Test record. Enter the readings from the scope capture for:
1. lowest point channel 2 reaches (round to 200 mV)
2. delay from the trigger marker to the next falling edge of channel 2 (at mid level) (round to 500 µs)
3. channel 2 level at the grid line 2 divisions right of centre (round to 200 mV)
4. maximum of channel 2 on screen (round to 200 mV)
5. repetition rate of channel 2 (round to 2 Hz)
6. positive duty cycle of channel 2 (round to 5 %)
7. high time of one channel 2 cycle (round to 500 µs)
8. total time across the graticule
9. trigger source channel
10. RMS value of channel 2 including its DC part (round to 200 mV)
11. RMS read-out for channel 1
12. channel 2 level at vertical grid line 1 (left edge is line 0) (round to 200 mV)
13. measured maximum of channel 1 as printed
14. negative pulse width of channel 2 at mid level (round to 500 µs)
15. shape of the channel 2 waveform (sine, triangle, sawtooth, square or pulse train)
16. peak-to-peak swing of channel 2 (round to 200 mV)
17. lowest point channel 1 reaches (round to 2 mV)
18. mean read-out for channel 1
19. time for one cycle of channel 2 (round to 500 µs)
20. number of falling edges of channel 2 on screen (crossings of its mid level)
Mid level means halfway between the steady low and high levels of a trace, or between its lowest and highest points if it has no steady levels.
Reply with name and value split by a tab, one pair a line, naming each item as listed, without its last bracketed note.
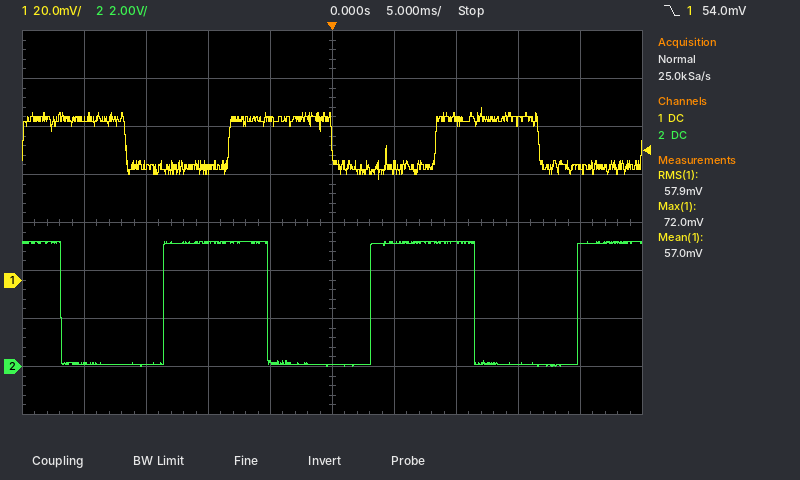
lowest point channel 2 reaches	0.0 V
delay from the trigger marker to the next falling edge of channel 2 (at mid level)	11.5 ms
channel 2 level at the grid line 2 divisions right of centre	5.2 V
maximum of channel 2 on screen	5.2 V
repetition rate of channel 2	60 Hz
positive duty cycle of channel 2	50 %
high time of one channel 2 cycle	8.5 ms
total time across the graticule	50 ms
trigger source channel	channel 1
RMS value of channel 2 including its DC part	3.6 V
RMS read-out for channel 1	57.9 mV
channel 2 level at vertical grid line 1 (left edge is line 0)	200 mV
measured maximum of channel 1 as printed	72.0 mV
negative pulse width of channel 2 at mid level	8.5 ms
shape of the channel 2 waveform	square
peak-to-peak swing of channel 2	5.2 V
lowest point channel 1 reaches	42 mV
mean read-out for channel 1	57.0 mV
time for one cycle of channel 2	16.5 ms
number of falling edges of channel 2 on screen	3
